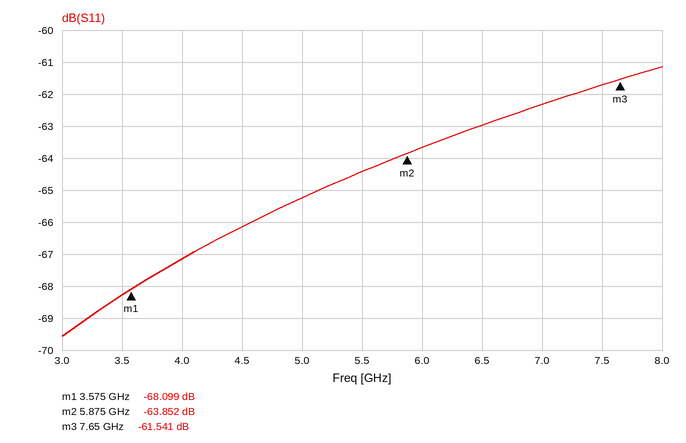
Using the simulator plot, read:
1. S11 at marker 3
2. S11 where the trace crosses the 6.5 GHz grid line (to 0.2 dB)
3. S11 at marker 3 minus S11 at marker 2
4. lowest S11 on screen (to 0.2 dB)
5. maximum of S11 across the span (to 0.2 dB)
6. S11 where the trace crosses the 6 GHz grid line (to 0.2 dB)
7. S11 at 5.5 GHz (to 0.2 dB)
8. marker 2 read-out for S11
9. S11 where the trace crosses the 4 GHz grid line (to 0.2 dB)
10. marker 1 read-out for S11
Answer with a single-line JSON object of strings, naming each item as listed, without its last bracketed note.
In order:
{"S11 at marker 3": "-61.541 dB", "S11 where the trace crosses the 6.5 GHz grid line": "-63.0 dB", "S11 at marker 3 minus S11 at marker 2": "2.311 dB", "lowest S11 on screen": "-69.6 dB", "maximum of S11 across the span": "-61.2 dB", "S11 where the trace crosses the 6 GHz grid line": "-63.6 dB", "S11 at 5.5 GHz": "-64.4 dB", "marker 2 read-out for S11": "-63.852 dB", "S11 where the trace crosses the 4 GHz grid line": "-67.2 dB", "marker 1 read-out for S11": "-68.099 dB"}
